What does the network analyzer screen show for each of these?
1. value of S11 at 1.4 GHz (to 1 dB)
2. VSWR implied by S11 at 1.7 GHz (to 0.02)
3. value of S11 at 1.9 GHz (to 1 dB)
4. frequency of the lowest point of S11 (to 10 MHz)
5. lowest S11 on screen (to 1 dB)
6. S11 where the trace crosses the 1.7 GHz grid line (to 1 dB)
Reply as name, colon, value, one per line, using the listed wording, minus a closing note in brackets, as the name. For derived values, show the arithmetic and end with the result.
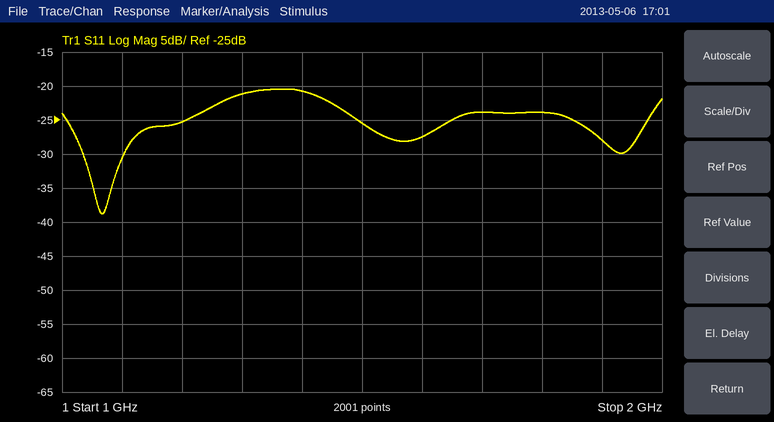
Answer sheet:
value of S11 at 1.4 GHz: -21 dB
VSWR implied by S11 at 1.7 GHz: |Γ| = 10^(-24/20) = 0.0631; VSWR = (1 + 0.0631)/(1 − 0.0631) ≈ 1.13, so 1.14 to the nearest 0.02
value of S11 at 1.9 GHz: -28 dB
frequency of the lowest point of S11: 1.07 GHz
lowest S11 on screen: -39 dB
S11 where the trace crosses the 1.7 GHz grid line: -24 dB
